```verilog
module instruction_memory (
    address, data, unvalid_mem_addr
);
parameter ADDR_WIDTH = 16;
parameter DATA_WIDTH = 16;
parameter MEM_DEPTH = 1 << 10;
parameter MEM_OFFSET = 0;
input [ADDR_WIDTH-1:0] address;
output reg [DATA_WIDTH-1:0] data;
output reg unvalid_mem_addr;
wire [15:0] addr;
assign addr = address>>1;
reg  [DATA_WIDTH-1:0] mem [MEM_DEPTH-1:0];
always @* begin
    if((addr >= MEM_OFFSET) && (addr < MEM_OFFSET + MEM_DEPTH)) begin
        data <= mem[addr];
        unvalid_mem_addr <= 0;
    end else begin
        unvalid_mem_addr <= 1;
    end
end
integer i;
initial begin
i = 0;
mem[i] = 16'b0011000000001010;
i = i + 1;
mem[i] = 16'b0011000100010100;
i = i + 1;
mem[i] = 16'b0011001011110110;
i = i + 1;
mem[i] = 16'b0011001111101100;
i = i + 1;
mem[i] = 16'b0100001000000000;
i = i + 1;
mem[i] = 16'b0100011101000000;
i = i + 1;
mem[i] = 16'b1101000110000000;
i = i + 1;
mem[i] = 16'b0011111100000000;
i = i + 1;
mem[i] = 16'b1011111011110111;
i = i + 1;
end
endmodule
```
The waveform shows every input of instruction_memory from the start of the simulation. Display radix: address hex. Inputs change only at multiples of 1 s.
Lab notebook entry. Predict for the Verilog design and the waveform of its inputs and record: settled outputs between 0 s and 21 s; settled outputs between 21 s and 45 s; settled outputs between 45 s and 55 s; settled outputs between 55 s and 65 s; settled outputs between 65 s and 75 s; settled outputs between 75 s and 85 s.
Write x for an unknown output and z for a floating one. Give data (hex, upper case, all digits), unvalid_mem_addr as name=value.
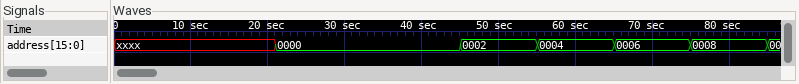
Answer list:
data=x, unvalid_mem_addr=1
data=300A, unvalid_mem_addr=0
data=3114, unvalid_mem_addr=0
data=32F6, unvalid_mem_addr=0
data=33EC, unvalid_mem_addr=0
data=4200, unvalid_mem_addr=0
